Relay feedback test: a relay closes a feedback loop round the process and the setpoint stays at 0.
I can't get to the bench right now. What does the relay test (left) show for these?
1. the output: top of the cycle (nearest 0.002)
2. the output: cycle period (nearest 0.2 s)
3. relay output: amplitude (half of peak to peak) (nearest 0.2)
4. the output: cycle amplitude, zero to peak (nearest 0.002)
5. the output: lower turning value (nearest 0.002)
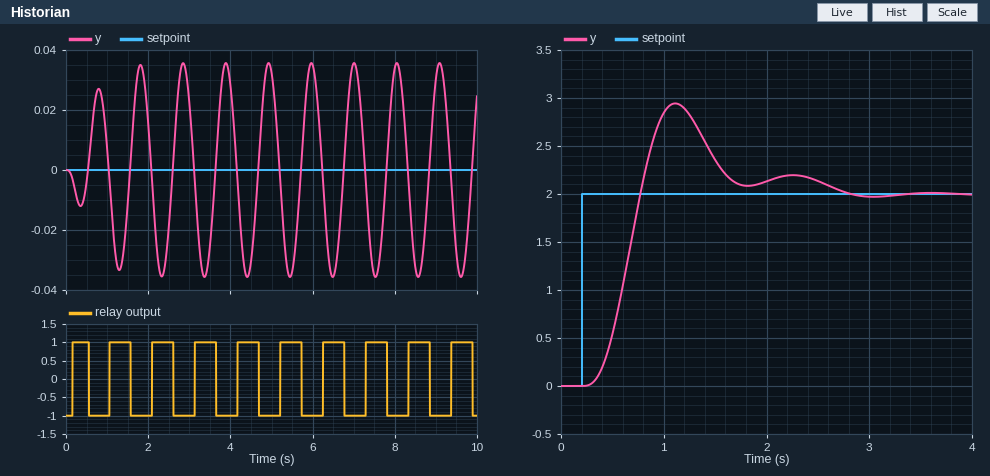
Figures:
0.036
1.0 s
1.0
0.036
-0.036
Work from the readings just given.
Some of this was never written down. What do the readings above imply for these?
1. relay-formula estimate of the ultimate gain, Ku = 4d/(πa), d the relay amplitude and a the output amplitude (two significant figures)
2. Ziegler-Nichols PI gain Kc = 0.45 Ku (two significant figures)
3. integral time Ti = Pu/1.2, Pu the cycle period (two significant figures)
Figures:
35
16
0.83 s
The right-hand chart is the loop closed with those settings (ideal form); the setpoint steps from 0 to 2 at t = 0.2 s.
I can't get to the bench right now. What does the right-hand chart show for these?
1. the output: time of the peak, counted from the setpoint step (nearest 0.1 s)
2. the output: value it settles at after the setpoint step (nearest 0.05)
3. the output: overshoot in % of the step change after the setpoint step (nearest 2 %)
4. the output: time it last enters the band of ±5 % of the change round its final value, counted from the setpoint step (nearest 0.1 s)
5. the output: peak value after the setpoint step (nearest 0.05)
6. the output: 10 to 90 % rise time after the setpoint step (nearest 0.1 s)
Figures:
0.9 s
2.00
48 %
2.4 s
2.95
0.3 s
